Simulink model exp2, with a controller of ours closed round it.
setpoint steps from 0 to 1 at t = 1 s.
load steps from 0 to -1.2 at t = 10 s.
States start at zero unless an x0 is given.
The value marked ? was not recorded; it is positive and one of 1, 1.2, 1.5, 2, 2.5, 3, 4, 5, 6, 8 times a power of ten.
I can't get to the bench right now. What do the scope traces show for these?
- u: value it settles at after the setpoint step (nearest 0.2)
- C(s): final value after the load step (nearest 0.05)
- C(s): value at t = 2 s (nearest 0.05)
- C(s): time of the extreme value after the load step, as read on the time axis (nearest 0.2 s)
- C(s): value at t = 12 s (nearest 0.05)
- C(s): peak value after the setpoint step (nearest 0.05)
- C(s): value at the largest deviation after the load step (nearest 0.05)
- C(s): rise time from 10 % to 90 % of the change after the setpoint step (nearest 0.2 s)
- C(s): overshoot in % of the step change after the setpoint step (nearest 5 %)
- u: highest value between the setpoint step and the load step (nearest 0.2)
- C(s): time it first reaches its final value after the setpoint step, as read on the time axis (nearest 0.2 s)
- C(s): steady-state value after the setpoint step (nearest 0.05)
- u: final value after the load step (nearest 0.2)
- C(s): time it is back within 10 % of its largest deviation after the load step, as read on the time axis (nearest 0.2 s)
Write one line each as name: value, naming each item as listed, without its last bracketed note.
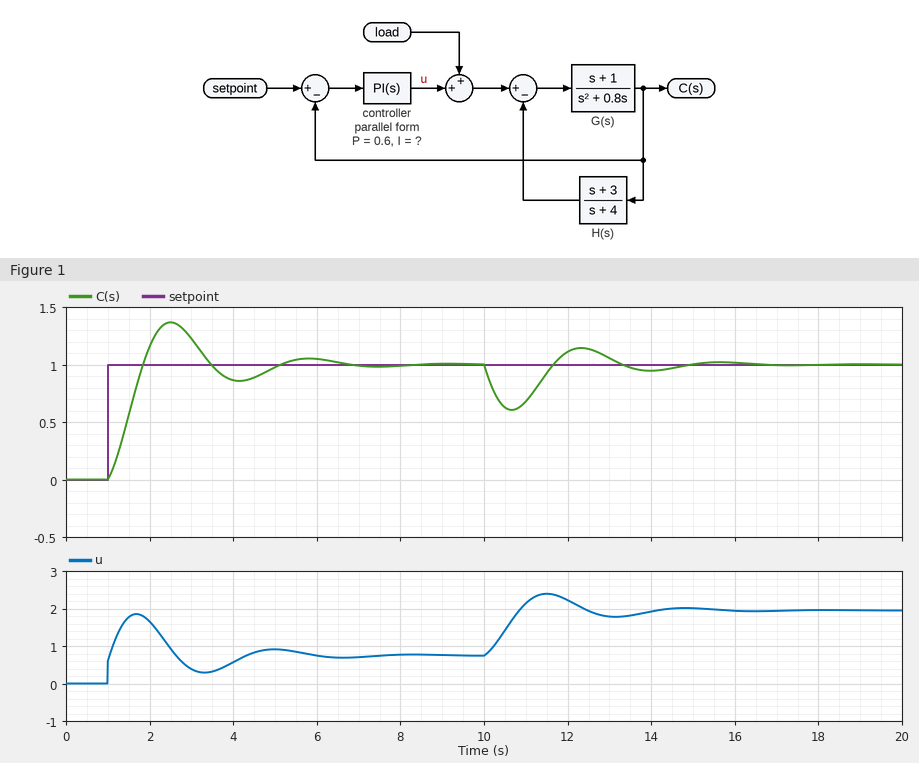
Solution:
u: value it settles at after the setpoint step: 0.8
C(s): final value after the load step: 1.00
C(s): value at t = 2 s: 1.15
C(s): time of the extreme value after the load step, as read on the time axis: 10.6 s
C(s): value at t = 12 s: 1.10
C(s): peak value after the setpoint step: 1.35
C(s): value at the largest deviation after the load step: 0.60
C(s): rise time from 10 % to 90 % of the change after the setpoint step: 0.6 s
C(s): overshoot in % of the step change after the setpoint step: 35 %
u: highest value between the setpoint step and the load step: 1.8
C(s): time it first reaches its final value after the setpoint step, as read on the time axis: 1.8 s
C(s): steady-state value after the setpoint step: 1.00
u: final value after the load step: 2.0
C(s): time it is back within 10 % of its largest deviation after the load step, as read on the time axis: 14.4 s
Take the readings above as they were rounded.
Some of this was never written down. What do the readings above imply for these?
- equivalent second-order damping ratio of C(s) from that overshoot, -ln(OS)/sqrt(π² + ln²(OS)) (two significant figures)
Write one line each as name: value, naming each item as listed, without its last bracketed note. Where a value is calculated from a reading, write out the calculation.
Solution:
equivalent second-order damping ratio of C(s) from that overshoot, -ln(OS)/sqrt(π² + ln²(OS)): ln(0.35) = -1.050; 1.050 / sqrt(9.870 + 1.102) = 0.32
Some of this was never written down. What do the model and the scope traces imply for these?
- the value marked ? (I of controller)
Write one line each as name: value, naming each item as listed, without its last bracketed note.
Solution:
the value marked ?: 4
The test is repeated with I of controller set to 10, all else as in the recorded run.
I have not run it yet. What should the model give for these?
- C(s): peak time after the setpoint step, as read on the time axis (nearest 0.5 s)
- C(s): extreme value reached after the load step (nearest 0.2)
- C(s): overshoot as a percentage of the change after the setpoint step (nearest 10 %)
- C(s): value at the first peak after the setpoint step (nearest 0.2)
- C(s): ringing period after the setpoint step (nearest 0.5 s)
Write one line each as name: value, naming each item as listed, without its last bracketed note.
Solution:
C(s): peak time after the setpoint step, as read on the time axis: 2.0 s
C(s): extreme value reached after the load step: 0.8
C(s): overshoot as a percentage of the change after the setpoint step: 50 %
C(s): value at the first peak after the setpoint step: 1.6
C(s): ringing period after the setpoint step: 2.0 s
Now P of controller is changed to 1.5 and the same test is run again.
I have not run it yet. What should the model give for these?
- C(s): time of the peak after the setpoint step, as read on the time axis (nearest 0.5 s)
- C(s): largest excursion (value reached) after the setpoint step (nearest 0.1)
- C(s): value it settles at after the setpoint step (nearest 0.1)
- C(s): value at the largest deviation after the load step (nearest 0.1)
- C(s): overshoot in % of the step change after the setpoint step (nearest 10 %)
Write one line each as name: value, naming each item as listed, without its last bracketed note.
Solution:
C(s): time of the peak after the setpoint step, as read on the time axis: 2.5 s
C(s): largest excursion (value reached) after the setpoint step: 1.2
C(s): value it settles at after the setpoint step: 1.0
C(s): value at the largest deviation after the load step: 0.7
C(s): overshoot in % of the step change after the setpoint step: 20 %
